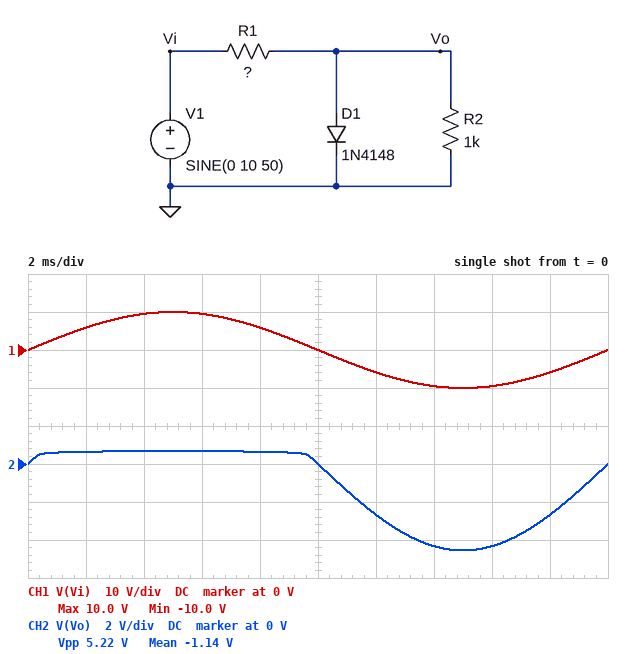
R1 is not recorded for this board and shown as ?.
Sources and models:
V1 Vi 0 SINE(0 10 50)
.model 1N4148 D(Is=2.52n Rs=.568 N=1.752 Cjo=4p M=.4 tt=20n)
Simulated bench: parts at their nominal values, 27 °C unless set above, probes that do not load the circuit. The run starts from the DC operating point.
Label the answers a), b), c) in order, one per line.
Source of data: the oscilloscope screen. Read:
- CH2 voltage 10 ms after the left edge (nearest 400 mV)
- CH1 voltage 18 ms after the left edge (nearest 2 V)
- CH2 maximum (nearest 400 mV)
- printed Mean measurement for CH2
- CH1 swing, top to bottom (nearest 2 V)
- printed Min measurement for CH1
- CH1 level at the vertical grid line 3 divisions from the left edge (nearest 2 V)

a) 0 V
b) -6 V
c) 800 mV
d) -1.14 V
e) 20 V
f) -10.0 V
g) 10 V
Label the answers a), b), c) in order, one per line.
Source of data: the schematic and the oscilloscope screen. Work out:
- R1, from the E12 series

a) 1.2 kΩ
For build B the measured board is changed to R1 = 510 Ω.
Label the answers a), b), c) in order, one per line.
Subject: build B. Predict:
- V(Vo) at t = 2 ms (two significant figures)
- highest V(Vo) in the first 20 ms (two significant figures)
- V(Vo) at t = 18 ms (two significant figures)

a) 690 mV
b) 720 mV
c) -3.9 V
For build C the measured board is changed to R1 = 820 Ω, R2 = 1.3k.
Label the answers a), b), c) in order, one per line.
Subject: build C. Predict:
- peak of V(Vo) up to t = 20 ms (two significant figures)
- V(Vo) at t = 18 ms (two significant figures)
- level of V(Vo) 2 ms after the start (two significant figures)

a) 700 mV
b) -3.6 V
c) 670 mV
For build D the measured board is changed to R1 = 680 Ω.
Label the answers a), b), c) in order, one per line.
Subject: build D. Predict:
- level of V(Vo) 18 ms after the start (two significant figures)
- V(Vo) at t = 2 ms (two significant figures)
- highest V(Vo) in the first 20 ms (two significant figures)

a) -3.5 V
b) 680 mV
c) 710 mV
